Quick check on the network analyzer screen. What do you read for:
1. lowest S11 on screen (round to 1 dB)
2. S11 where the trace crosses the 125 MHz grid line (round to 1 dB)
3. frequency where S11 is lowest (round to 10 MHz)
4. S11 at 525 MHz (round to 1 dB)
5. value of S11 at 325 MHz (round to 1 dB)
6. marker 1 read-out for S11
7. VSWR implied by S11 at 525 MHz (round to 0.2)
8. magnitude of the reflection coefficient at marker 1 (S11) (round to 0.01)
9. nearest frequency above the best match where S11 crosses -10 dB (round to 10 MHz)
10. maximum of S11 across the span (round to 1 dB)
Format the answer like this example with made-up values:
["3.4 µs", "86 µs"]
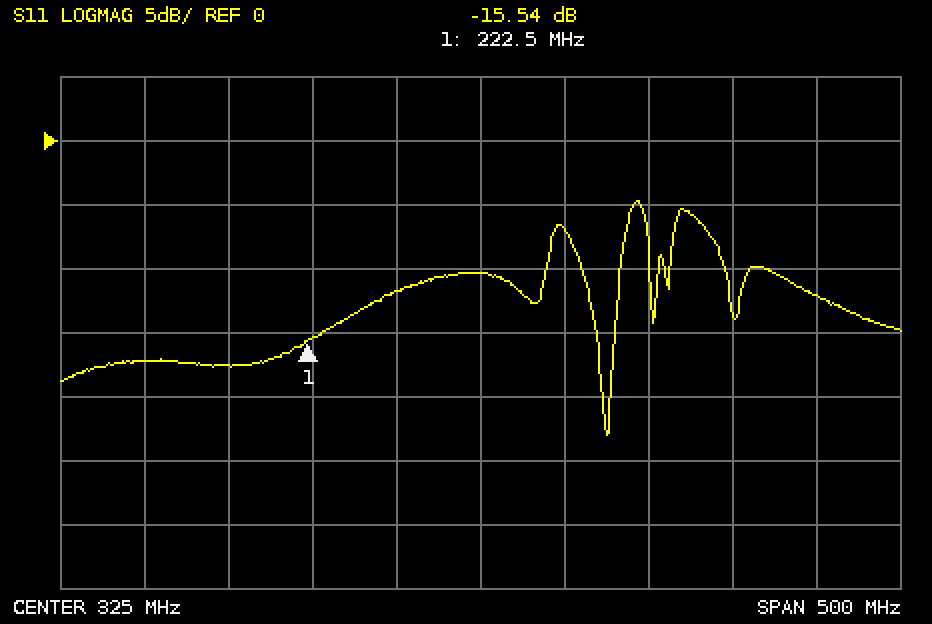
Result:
["-23 dB", "-17 dB", "400 MHz", "-12 dB", "-10 dB", "-15.54 dB", "1.6", "0.17", "410 MHz", "-5 dB"]
